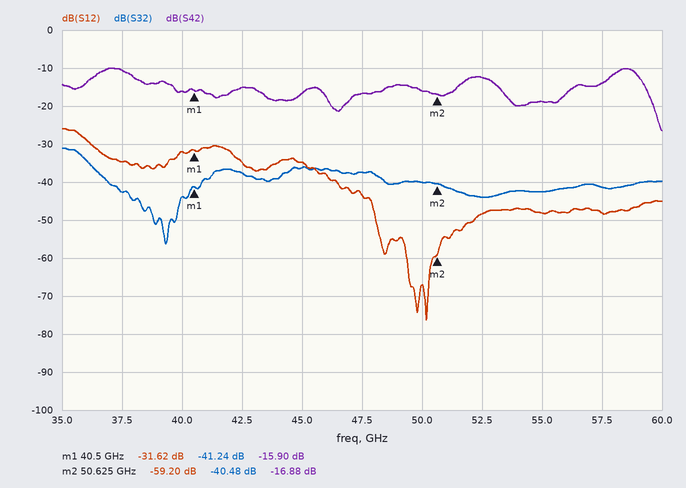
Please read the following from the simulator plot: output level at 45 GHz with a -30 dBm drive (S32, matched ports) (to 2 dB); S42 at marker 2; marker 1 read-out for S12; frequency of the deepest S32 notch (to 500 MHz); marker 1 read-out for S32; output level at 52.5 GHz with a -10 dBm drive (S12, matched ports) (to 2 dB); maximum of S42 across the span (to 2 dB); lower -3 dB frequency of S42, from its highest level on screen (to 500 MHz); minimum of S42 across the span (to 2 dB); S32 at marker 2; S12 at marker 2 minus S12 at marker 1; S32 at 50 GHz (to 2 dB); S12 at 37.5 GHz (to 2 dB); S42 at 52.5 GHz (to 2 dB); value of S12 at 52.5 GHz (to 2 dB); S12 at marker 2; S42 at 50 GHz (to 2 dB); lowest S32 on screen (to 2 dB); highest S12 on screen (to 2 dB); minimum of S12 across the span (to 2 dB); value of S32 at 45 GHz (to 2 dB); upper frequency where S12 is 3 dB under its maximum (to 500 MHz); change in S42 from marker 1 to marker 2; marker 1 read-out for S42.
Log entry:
-66 dBm
-16.88 dB
-31.62 dB
39.5 GHz
-41.24 dB
-58 dBm
-10 dB
36.0 GHz
-26 dB
-40.48 dB
-27.58 dB
-40 dB
-34 dB
-12 dB
-48 dB
-59.20 dB
-16 dB
-56 dB
-26 dB
-76 dB
-36 dB
36.0 GHz
-0.98 dB
-15.90 dB
